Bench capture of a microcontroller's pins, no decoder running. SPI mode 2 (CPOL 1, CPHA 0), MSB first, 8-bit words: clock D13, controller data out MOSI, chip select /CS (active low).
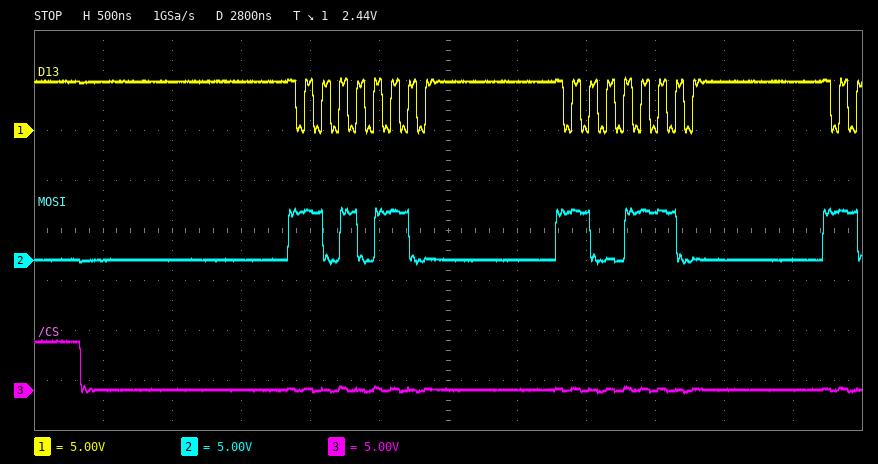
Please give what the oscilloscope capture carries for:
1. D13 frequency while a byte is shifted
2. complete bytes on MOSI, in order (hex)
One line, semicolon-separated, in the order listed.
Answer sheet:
8 MHz; D6 CE
